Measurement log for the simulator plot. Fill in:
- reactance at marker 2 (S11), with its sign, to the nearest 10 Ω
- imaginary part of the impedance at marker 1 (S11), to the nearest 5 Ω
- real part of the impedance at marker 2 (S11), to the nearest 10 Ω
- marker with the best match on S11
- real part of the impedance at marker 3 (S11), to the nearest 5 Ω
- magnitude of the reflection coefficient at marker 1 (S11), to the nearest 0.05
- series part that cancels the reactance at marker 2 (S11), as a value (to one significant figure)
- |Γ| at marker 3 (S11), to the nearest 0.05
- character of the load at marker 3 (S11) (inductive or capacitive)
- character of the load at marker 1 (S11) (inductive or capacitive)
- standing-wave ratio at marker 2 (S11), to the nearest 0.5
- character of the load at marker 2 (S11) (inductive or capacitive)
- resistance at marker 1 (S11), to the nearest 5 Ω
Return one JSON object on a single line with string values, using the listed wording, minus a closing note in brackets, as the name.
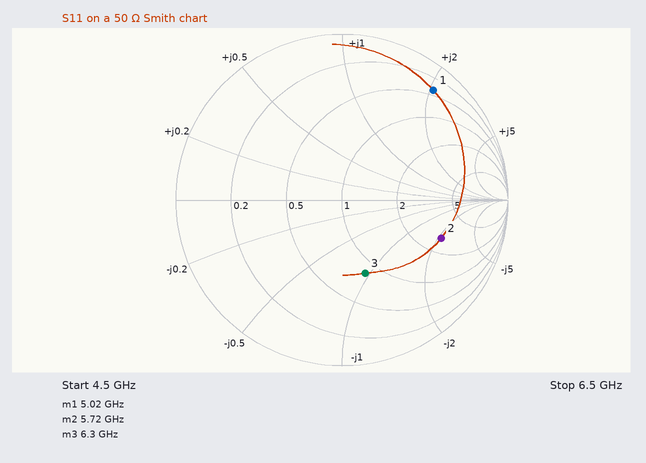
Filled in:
{"reactance at marker 2 (S11), with its sign, to the nearest 10 Ω": "-110 Ω", "imaginary part of the impedance at marker 1 (S11), to the nearest 5 Ω": "+105 Ω", "real part of the impedance at marker 2 (S11), to the nearest 10 Ω": "140 Ω", "marker with the best match on S11": "marker 3", "real part of the impedance at marker 3 (S11), to the nearest 5 Ω": "40 Ω", "magnitude of the reflection coefficient at marker 1 (S11), to the nearest 0.05": "0.85", "series part that cancels the reactance at marker 2 (S11), as a value": "3 nH", "|Γ| at marker 3 (S11), to the nearest 0.05": "0.45", "character of the load at marker 3 (S11)": "capacitive", "character of the load at marker 1 (S11)": "inductive", "standing-wave ratio at marker 2 (S11), to the nearest 0.5": "4.5", "character of the load at marker 2 (S11)": "capacitive", "resistance at marker 1 (S11), to the nearest 5 Ω": "20 Ω"}
